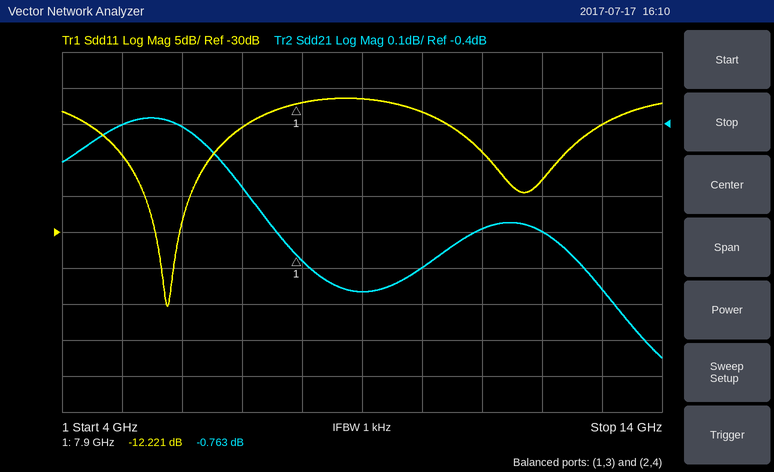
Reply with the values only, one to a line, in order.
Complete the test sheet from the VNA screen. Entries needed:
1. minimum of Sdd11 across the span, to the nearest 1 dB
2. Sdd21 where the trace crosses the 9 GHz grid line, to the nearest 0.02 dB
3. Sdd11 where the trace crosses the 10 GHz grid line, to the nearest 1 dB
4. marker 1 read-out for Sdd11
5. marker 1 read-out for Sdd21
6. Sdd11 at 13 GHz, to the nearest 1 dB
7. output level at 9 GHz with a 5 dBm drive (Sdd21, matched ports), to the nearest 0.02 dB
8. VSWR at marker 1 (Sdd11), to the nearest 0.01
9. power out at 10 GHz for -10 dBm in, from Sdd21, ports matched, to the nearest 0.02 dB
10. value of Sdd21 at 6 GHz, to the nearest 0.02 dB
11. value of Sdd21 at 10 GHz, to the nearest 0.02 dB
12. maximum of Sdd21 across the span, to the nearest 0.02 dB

-40 dB
-0.86 dB
-13 dB
-12.221 dB
-0.763 dB
-15 dB
4.14 dBm
1.65
-10.80 dBm
-0.40 dB
-0.80 dB
-0.38 dB
